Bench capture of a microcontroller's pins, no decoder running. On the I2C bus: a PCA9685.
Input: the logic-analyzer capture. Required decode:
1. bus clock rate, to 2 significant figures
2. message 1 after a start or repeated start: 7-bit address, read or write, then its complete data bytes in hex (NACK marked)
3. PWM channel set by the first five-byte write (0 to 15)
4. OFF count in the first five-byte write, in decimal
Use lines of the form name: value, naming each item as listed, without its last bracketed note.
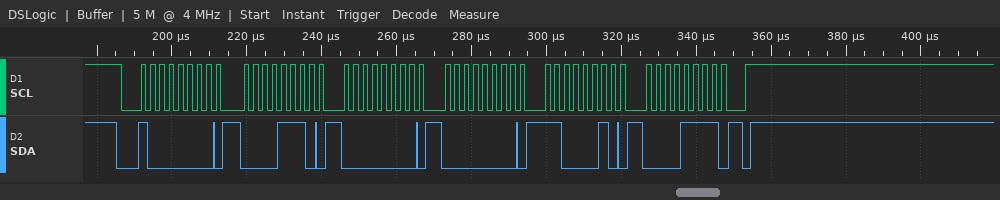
bus clock rate, to 2 significant figures: 400 kHz
message 1 after a start or repeated start: 7-bit address, read or write, then its complete data bytes in hex: 0x40 write: 0E 00 00 C2 0F
PWM channel set by the first five-byte write: 2
OFF count in the first five-byte write, in decimal: 4034
